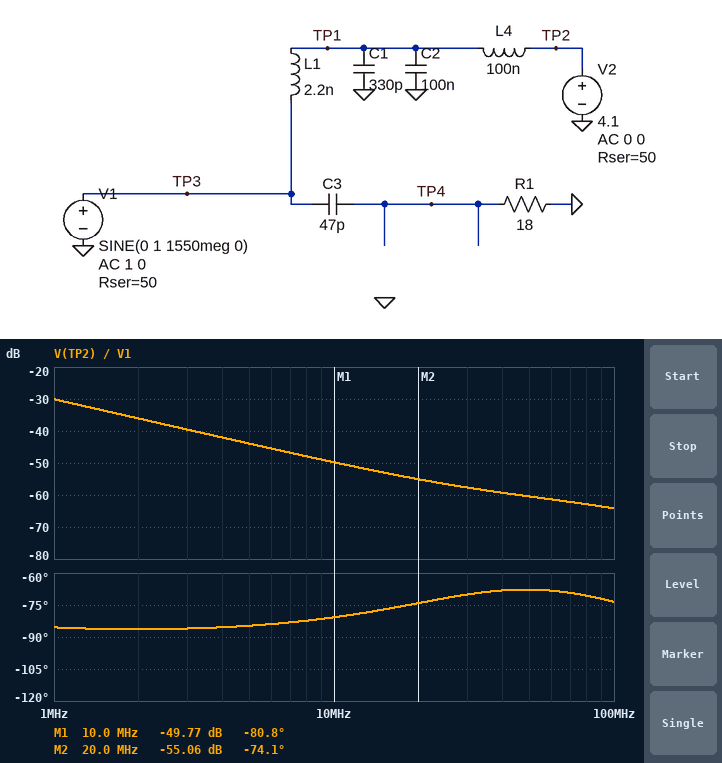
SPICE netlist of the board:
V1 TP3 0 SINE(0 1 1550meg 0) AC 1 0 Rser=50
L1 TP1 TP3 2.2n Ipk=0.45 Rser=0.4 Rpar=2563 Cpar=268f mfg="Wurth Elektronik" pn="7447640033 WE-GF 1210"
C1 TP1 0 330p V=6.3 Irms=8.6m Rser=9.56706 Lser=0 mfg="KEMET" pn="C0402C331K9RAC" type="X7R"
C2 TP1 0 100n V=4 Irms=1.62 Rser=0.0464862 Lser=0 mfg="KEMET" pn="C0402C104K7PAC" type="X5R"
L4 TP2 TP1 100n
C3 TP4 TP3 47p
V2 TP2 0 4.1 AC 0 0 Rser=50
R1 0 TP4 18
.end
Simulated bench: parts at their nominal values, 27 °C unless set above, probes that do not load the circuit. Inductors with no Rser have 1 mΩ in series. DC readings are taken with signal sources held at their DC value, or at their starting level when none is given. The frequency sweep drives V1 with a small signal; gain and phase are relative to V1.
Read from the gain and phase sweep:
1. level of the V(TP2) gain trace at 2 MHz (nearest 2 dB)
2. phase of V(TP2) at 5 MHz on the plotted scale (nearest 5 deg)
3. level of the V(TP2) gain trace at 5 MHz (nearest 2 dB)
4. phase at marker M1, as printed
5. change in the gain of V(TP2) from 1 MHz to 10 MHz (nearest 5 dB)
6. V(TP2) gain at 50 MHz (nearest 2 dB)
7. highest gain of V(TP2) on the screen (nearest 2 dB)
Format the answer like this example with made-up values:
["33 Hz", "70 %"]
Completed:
["-36 dB", "-85 deg", "-44 dB", "-80.8 deg", "-20 dB", "-60 dB", "-30 dB"]
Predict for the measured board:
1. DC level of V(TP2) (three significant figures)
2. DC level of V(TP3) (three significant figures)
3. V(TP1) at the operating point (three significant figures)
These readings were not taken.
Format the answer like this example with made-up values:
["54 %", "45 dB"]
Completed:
["2.06 V", "2.04 V", "2.06 V"]
